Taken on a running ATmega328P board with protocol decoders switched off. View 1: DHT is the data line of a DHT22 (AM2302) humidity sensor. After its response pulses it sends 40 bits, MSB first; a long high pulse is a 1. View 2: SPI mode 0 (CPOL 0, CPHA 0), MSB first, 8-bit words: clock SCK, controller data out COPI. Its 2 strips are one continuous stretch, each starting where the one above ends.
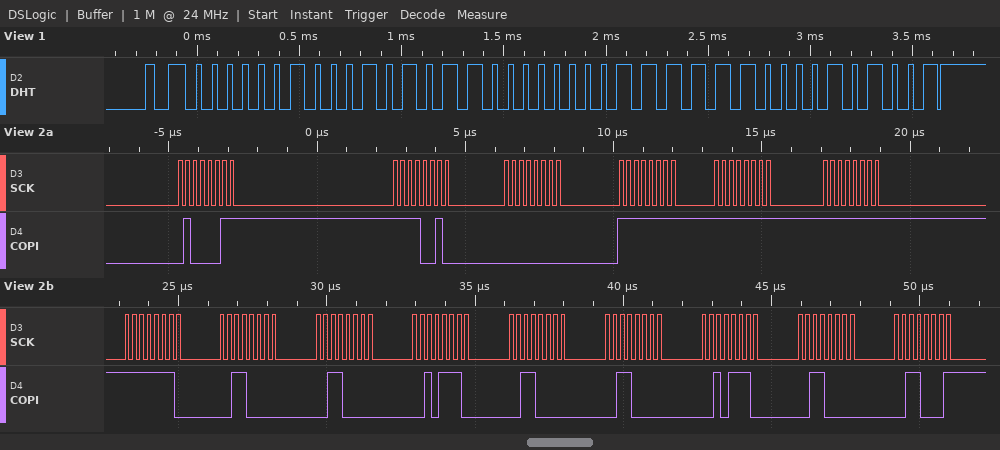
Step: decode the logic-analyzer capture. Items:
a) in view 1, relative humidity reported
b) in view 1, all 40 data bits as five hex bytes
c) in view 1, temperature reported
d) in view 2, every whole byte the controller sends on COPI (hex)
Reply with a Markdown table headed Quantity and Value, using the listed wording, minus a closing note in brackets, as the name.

| Quantity | Value |
|---|---|
| in view 1, relative humidity reported | 55.5 % |
| in view 1, all 40 data bits as five hex bytes | 02 2B 00 FC 29 |
| in view 1, temperature reported | 25.2 °C |
| in view 2, every whole byte the controller sends on COPI | 43 F2 00 FF FF FF FE 30 30 2E 30 30 2E 30 31 |
